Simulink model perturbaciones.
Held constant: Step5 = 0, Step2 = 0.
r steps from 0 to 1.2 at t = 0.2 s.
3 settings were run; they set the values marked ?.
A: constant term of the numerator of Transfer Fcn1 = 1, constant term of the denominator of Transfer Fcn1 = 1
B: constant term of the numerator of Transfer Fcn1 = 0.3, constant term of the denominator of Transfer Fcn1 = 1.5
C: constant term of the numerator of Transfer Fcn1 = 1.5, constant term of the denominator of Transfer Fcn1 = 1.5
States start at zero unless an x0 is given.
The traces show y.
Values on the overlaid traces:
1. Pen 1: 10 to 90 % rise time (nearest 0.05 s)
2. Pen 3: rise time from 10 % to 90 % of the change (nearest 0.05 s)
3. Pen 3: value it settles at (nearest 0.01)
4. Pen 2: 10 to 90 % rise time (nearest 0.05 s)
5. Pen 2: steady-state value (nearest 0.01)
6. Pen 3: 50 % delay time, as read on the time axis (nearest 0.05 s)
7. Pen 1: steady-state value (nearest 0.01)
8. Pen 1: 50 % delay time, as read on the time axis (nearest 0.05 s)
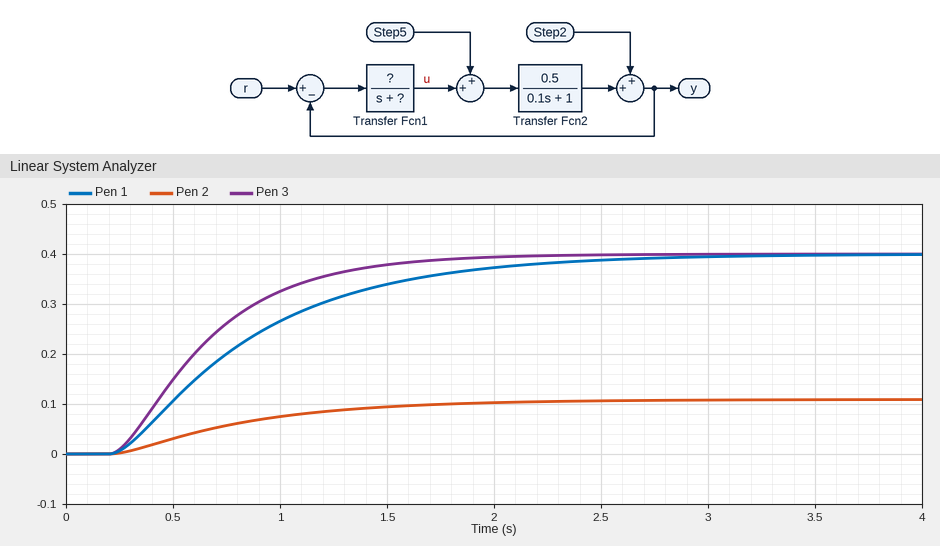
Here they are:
1.40 s
0.95 s
0.40
1.35 s
0.11
0.60 s
0.40
0.75 s
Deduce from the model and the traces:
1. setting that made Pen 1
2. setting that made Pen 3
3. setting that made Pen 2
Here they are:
A
C
B
